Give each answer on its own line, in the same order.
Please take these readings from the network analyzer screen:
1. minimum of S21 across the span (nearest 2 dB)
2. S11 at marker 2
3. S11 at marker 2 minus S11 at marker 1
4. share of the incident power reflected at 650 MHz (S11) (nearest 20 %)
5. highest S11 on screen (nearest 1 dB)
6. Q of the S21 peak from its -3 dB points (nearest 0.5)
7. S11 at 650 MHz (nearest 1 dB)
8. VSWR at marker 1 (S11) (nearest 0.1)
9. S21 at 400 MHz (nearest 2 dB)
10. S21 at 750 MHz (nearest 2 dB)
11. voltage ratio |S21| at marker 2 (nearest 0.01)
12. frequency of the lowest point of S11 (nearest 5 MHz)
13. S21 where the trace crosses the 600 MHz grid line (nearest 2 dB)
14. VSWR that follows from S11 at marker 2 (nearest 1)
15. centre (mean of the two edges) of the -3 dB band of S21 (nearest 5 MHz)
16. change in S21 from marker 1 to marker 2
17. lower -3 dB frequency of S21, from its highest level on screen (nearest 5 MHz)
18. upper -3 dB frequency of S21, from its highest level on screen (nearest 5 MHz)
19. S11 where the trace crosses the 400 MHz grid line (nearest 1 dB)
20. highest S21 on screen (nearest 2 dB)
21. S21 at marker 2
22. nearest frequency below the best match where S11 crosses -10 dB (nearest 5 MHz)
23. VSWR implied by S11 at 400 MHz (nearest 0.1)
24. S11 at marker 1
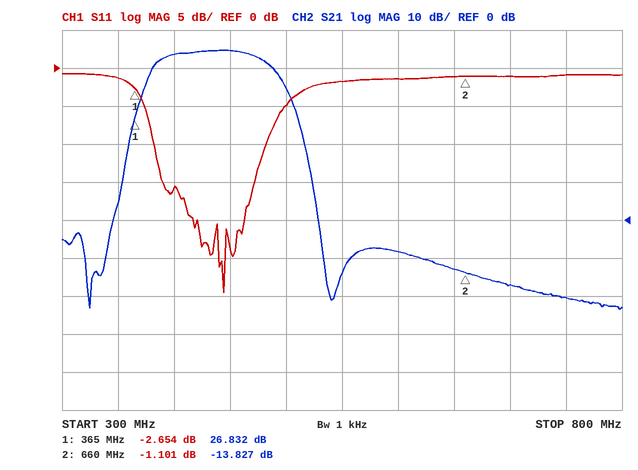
-24 dB
-1.101 dB
1.553 dB
80 %
-1 dB
4.5
-1 dB
6.6
44 dB
-20 dB
0.20
445 MHz
-8 dB
16
435 MHz
-40.659 dB
385 MHz
480 MHz
-16 dB
44 dB
-13.827 dB
380 MHz
1.4
-2.654 dB
